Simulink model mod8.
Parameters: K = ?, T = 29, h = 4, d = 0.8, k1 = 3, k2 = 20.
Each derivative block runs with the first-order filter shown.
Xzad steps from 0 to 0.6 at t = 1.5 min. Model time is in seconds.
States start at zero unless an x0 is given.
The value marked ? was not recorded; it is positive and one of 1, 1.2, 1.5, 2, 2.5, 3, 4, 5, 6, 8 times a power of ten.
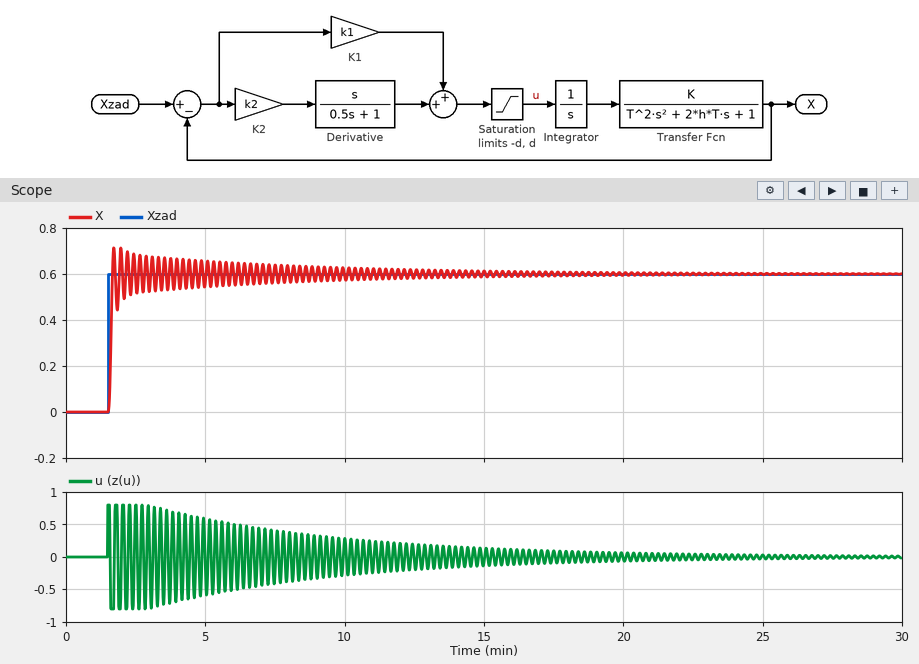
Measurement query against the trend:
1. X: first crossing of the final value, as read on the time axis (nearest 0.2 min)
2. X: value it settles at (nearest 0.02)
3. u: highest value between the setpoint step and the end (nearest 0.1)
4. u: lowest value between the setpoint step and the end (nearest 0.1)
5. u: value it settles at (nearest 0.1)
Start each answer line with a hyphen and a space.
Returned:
- 1.6 min
- 0.60
- 0.8
- -0.8
- 0.0
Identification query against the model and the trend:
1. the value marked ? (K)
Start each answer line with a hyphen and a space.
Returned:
- 10
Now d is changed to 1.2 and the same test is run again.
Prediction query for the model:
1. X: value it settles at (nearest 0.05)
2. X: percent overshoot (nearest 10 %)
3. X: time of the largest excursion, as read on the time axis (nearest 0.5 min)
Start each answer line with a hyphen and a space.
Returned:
- 0.60
- 20 %
- 2.0 min
